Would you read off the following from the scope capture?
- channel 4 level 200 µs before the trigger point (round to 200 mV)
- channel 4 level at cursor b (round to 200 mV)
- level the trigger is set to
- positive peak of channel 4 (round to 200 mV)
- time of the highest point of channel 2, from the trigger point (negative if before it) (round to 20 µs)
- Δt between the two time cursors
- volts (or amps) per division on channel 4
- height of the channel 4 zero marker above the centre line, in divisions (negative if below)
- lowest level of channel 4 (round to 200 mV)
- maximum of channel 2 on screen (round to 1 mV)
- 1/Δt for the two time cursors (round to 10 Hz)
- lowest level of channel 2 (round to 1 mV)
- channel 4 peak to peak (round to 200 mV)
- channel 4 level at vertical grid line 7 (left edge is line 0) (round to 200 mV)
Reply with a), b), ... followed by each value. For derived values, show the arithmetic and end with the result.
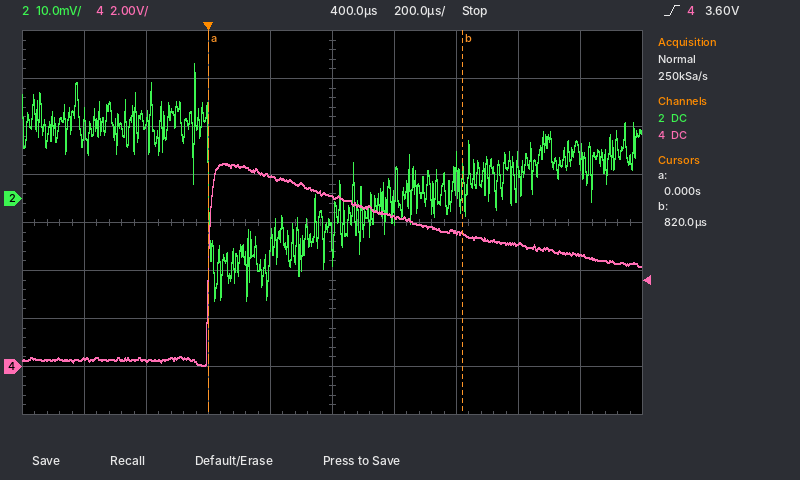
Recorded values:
a) 200 mV
b) 5.6 V
c) 3.60 V
d) 8.4 V
e) -40 µs
f) 820 µs − (0 s) = 820 µs
g) 2 V
h) -3.0 div
i) 0.0 V
j) 28 mV
k) 1 / 820 µs ≈ 1.22 kHz
l) -21 mV
m) 8.4 V − (0.0 V) = 8.4 V
n) 5.6 V
